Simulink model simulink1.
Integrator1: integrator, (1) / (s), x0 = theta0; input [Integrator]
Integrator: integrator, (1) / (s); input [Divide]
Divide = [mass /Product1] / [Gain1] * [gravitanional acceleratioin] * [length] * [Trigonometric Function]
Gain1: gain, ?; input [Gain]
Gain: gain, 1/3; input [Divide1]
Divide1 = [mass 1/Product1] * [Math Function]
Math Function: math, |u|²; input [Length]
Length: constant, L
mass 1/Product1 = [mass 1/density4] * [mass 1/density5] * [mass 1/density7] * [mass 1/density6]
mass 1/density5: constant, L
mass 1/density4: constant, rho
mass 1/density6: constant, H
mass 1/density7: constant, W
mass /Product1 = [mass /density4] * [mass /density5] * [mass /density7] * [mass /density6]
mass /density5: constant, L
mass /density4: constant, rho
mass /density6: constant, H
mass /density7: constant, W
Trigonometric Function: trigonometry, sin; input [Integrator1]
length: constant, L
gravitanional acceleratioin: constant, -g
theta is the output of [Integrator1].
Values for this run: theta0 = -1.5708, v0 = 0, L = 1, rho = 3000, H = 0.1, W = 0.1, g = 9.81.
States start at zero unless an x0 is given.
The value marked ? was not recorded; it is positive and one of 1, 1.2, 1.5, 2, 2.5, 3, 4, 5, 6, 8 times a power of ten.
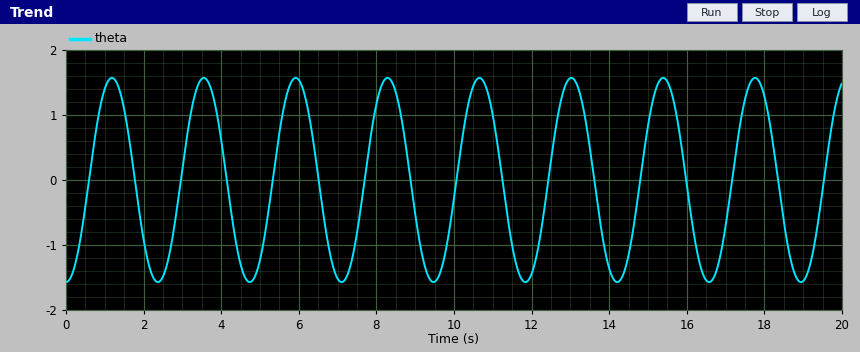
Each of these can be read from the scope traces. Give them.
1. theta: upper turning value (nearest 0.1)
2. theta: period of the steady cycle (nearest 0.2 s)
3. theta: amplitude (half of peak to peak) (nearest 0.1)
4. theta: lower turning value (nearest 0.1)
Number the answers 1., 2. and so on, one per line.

1. 1.6
2. 2.4 s
3. 1.6
4. -1.6
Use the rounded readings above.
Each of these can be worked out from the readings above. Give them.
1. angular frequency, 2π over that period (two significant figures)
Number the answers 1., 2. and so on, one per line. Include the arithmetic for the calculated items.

1. 2π / 2.4 = 2.6 rad/s
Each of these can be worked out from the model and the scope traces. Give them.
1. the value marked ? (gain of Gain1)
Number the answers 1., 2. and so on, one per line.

1. 3
